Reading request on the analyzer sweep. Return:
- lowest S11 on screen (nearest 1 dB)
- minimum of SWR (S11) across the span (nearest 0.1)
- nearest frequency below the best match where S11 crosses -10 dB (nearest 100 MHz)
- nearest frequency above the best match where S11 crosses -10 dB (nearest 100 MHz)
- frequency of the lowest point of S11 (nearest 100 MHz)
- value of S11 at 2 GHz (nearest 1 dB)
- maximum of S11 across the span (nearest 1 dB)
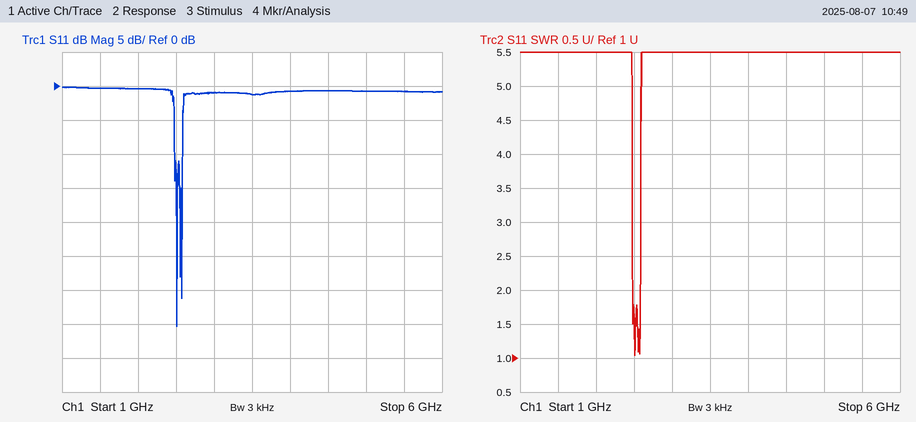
-35 dB
1.0
2.5 GHz
2.6 GHz
2.5 GHz
0 dB
0 dB
